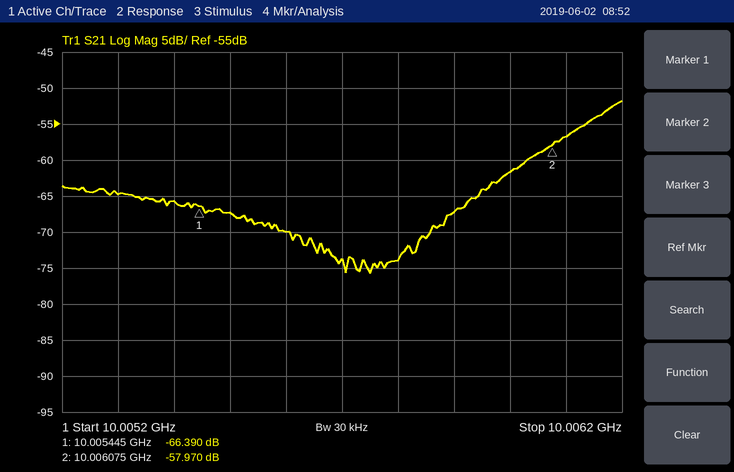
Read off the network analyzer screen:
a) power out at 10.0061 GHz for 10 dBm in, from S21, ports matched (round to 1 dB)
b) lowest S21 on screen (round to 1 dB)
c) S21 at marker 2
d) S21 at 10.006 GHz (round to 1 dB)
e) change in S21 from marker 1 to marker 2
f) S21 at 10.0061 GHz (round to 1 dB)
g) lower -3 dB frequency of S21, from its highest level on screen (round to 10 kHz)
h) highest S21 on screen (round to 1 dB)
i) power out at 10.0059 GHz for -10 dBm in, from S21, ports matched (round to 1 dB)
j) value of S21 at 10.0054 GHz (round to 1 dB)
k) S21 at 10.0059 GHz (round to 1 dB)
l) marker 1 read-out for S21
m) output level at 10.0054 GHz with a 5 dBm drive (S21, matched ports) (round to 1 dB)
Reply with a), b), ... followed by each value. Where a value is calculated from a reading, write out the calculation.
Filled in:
a) 10 dBm + (-57 dB) = -47 dBm
b) -76 dB
c) -57.970 dB
d) -62 dB
e) -57.97 − (-66.39) = 8.420 dB
f) -57 dB
g) 10.00614 GHz
h) -52 dB
i) -10 dBm + (-67 dB) = -77 dBm
j) -66 dB
k) -67 dB
l) -66.390 dB
m) 5 dBm + (-66 dB) = -61 dBm
